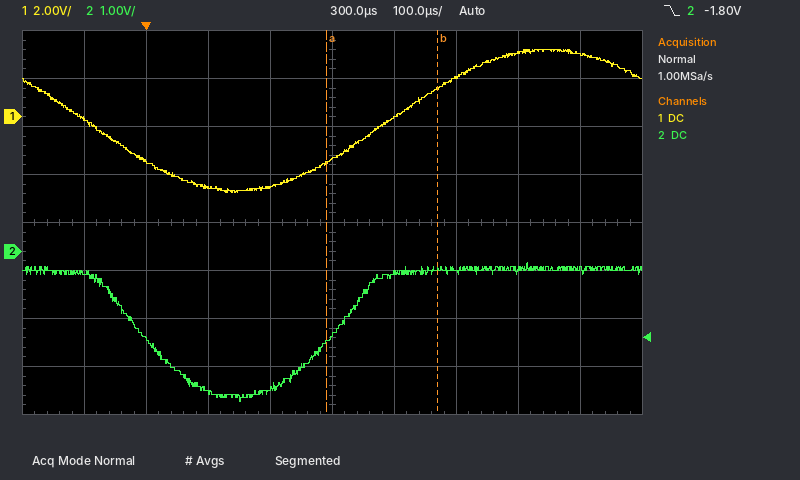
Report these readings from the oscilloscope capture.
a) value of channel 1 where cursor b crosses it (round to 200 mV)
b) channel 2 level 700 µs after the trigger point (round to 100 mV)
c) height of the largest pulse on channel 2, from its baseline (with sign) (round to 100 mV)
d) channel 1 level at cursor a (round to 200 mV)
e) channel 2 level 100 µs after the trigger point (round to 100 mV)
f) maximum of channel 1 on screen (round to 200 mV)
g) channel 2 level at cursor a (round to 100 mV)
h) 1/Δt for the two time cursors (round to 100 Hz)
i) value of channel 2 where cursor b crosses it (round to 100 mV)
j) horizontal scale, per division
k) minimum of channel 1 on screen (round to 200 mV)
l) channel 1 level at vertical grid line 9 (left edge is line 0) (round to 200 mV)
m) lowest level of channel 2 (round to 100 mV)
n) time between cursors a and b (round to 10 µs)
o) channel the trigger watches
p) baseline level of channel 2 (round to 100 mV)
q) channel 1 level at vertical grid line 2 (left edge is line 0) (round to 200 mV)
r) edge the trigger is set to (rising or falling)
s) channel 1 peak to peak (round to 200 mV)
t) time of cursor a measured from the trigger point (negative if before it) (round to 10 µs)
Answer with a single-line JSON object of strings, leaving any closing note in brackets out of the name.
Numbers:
{"value of channel 1 where cursor b crosses it": "1.2 V", "channel 2 level 700 µs after the trigger point": "-400 mV", "height of the largest pulse on channel 2, from its baseline (with sign)": "-2.7 V", "channel 1 level at cursor a": "-2.0 V", "channel 2 level 100 µs after the trigger point": "-2.9 V", "maximum of channel 1 on screen": "2.8 V", "channel 2 level at cursor a": "-1.9 V", "1/Δt for the two time cursors": "5.6 kHz", "value of channel 2 where cursor b crosses it": "-400 mV", "horizontal scale, per division": "100 µs", "minimum of channel 1 on screen": "-3.2 V", "channel 1 level at vertical grid line 9 (left edge is line 0)": "2.6 V", "lowest level of channel 2": "-3.1 V", "time between cursors a and b": "180 µs", "channel the trigger watches": "channel 2", "baseline level of channel 2": "-400 mV", "channel 1 level at vertical grid line 2 (left edge is line 0)": "-1.8 V", "edge the trigger is set to": "falling", "channel 1 peak to peak": "6.0 V", "time of cursor a measured from the trigger point (negative if before it)": "+290 µs"}
